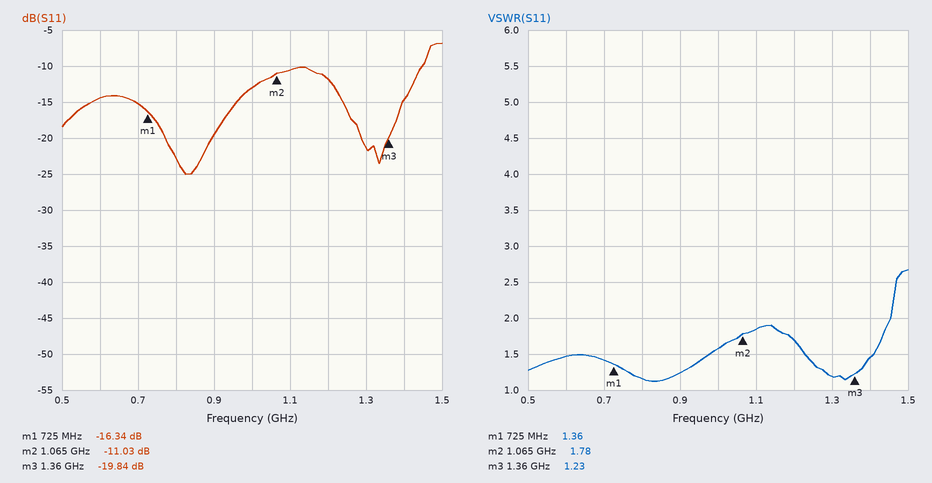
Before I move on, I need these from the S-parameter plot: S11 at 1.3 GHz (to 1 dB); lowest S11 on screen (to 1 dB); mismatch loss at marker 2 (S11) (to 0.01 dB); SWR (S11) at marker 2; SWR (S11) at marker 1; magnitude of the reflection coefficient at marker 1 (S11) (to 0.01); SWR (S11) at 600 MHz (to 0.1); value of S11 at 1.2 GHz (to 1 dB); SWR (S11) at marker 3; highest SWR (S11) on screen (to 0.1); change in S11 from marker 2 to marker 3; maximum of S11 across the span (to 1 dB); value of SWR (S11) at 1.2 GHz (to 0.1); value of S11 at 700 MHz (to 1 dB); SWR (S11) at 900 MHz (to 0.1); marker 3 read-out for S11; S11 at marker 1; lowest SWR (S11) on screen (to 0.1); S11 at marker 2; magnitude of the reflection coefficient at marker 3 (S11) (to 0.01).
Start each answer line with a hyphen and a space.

- -21 dB
- -25 dB
- 0.36 dB
- 1.78
- 1.36
- 0.15
- 1.5
- -12 dB
- 1.23
- 2.7
- -8.81 dB
- -7 dB
- 1.7
- -15 dB
- 1.2
- -19.84 dB
- -16.34 dB
- 1.1
- -11.03 dB
- 0.10
